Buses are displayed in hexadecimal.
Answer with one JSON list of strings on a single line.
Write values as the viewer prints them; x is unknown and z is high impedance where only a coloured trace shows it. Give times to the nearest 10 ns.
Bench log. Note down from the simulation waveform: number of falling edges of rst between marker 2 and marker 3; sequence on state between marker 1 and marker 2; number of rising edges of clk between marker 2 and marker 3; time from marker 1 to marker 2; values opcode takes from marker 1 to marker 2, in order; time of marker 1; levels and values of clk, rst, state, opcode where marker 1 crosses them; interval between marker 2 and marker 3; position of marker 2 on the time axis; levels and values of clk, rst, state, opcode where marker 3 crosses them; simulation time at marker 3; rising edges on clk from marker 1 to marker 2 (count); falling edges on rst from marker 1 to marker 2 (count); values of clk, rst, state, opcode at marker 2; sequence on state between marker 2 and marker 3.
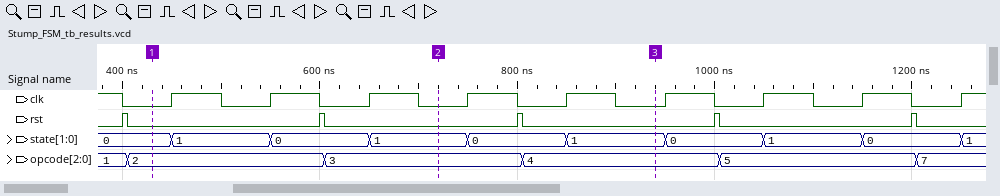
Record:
["1", "0, 1, 0, 1", "2", "290 ns", "2, 3", "430 ns", "clk=0, rst=0, state=0, opcode=2", "220 ns", "720 ns", "clk=0, rst=0, state=1, opcode=4", "940 ns", "3", "1", "clk=0, rst=0, state=1, opcode=3", "1, 0, 1"]
